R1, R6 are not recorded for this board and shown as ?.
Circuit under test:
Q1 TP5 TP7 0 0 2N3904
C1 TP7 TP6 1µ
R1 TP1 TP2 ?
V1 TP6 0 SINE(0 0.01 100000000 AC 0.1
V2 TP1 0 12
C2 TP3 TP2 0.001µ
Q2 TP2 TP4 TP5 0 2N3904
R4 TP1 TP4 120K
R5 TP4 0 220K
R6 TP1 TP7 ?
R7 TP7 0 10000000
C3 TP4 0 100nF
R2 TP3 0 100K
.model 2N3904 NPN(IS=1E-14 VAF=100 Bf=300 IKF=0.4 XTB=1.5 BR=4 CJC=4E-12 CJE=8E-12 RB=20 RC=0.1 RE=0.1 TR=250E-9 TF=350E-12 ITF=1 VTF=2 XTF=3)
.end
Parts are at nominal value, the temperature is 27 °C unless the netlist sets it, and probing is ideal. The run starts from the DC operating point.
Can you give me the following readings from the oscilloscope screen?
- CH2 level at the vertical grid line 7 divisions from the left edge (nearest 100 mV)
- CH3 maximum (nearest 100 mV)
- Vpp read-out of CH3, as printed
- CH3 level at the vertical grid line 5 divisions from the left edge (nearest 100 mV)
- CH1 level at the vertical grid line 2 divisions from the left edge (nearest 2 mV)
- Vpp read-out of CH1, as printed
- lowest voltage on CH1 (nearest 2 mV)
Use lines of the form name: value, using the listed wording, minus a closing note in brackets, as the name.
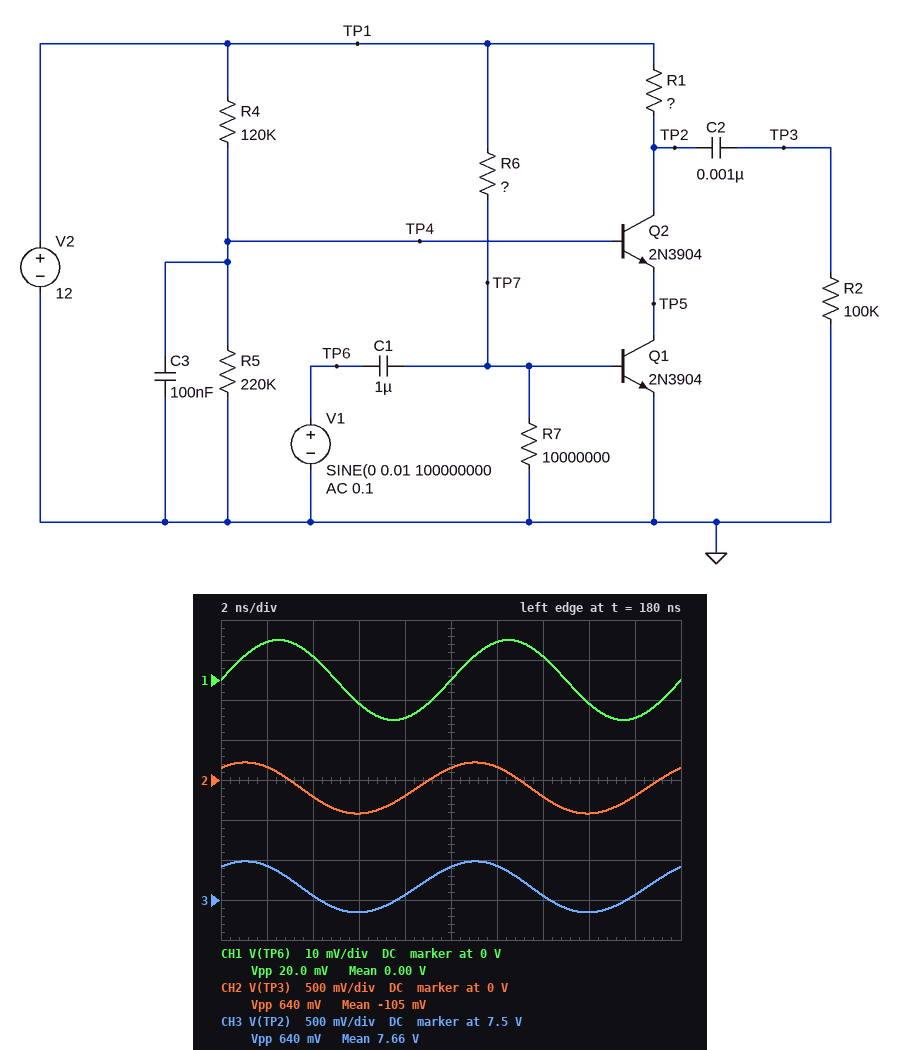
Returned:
CH2 level at the vertical grid line 7 divisions from the left edge: -200 mV
CH3 maximum: 8.0 V
Vpp read-out of CH3, as printed: 640 mV
CH3 level at the vertical grid line 5 divisions from the left edge: 7.9 V
CH1 level at the vertical grid line 2 divisions from the left edge: 6 mV
Vpp read-out of CH1, as printed: 20.0 mV
lowest voltage on CH1: -10 mV
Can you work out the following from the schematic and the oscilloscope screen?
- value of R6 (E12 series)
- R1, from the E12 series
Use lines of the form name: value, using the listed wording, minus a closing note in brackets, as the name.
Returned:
value of R6: 1.5 MΩ
R1, from the E12 series: 1.8 kΩ
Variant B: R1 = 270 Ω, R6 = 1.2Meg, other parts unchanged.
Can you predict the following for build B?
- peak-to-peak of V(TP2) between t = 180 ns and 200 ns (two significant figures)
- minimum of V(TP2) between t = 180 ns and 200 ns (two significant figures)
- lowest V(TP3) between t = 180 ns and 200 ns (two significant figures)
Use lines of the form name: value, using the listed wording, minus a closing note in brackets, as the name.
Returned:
peak-to-peak of V(TP2) between t = 180 ns and 200 ns: 440 mV
minimum of V(TP2) between t = 180 ns and 200 ns: 11 V
lowest V(TP3) between t = 180 ns and 200 ns: -250 mV
